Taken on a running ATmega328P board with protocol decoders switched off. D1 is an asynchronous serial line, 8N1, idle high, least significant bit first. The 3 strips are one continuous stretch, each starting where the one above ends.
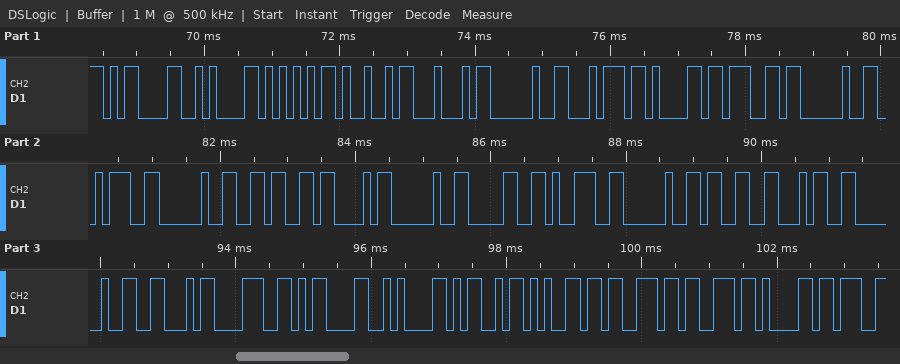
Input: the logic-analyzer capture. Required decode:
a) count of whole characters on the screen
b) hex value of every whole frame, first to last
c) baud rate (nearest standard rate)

30
0D 0A 55 49 44 20 74 61 67 20 3A 20 36 43 20 30 39 20 33 34 20 46 38 0D 0A 4D 65 73 73 61
9600 baud
